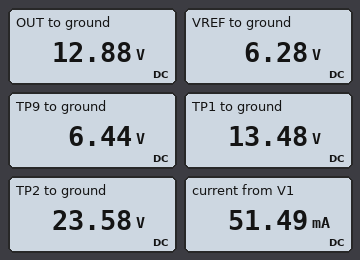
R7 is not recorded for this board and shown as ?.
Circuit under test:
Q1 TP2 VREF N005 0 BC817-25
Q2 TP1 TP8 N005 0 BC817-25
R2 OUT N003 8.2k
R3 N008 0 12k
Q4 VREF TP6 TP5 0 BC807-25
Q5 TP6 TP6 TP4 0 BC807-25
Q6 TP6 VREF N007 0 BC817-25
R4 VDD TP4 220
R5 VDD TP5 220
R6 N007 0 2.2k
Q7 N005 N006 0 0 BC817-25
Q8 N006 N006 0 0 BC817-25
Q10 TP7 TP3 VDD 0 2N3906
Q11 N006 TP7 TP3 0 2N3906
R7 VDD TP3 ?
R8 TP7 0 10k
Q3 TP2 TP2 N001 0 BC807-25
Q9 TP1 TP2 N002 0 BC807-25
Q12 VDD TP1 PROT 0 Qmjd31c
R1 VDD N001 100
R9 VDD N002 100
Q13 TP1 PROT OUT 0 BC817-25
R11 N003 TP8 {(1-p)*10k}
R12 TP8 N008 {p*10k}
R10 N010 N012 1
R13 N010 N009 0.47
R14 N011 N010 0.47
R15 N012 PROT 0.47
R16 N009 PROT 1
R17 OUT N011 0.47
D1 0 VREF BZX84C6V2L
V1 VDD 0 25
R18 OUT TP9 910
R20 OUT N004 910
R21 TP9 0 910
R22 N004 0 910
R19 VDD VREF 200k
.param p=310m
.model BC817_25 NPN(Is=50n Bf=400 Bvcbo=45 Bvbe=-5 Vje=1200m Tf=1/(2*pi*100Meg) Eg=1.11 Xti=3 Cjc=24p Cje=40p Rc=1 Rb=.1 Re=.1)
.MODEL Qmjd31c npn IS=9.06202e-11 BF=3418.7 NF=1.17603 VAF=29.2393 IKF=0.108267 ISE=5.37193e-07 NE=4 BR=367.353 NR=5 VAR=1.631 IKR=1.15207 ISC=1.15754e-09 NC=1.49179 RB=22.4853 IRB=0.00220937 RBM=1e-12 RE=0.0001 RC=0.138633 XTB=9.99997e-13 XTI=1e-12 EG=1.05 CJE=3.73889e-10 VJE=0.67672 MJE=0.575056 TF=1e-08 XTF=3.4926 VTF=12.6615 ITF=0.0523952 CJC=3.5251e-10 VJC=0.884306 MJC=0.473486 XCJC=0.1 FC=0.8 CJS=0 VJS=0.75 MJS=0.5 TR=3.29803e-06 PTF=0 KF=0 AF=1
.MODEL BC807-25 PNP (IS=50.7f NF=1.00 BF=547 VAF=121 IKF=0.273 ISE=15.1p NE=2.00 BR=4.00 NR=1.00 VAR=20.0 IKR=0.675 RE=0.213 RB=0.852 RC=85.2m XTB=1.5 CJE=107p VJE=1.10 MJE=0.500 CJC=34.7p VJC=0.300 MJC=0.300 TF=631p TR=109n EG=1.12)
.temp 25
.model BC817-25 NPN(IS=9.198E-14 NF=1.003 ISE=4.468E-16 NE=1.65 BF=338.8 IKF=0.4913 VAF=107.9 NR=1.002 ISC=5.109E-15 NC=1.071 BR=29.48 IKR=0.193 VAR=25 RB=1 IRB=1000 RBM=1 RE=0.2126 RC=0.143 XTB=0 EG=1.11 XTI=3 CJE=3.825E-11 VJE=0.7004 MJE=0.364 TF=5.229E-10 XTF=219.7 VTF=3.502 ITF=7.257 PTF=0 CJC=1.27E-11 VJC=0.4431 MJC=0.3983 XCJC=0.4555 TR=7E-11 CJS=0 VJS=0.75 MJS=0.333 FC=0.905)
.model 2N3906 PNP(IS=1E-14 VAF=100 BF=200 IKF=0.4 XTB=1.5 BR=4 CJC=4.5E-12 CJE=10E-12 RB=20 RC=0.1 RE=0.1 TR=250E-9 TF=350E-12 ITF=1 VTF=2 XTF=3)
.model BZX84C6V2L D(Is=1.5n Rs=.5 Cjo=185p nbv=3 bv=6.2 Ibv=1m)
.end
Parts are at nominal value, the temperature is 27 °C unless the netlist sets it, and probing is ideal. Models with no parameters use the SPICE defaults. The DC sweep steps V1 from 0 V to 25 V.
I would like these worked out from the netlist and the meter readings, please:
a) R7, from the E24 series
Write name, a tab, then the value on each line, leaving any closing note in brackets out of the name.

R7, from the E24 series	47 Ω
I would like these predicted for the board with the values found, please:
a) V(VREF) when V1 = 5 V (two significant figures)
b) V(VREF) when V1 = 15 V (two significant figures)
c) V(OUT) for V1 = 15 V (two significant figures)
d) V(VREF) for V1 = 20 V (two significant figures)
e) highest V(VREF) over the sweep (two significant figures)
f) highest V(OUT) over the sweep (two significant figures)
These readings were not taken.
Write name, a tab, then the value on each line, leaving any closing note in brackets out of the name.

V(VREF) when V1 = 5 V	4.4 V
V(VREF) when V1 = 15 V	6.3 V
V(OUT) for V1 = 15 V	13 V
V(VREF) for V1 = 20 V	6.3 V
highest V(VREF) over the sweep	6.3 V
highest V(OUT) over the sweep	13 V
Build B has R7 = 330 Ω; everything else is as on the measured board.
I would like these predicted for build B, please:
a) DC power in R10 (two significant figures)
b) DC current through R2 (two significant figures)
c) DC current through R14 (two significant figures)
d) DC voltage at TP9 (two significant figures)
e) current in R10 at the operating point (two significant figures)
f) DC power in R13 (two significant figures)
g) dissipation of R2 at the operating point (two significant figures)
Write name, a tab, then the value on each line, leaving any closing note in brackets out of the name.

DC power in R10	51 µW
DC current through R2	420 µA
DC current through R14	14 mA
DC voltage at TP9	6.3 V
current in R10 at the operating point	7.1 mA
DC power in R13	24 µW
dissipation of R2 at the operating point	1.4 mW
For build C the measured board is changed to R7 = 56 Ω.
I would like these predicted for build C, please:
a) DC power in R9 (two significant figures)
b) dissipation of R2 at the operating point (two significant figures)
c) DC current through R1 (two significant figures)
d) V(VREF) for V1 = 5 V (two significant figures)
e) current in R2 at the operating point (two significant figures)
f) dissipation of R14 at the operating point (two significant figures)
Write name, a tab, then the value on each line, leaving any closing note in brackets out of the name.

DC power in R9	4.0 mW
dissipation of R2 at the operating point	1.5 mW
DC current through R1	6.3 mA
V(VREF) for V1 = 5 V	4.5 V
current in R2 at the operating point	430 µA
dissipation of R14 at the operating point	99 µW
